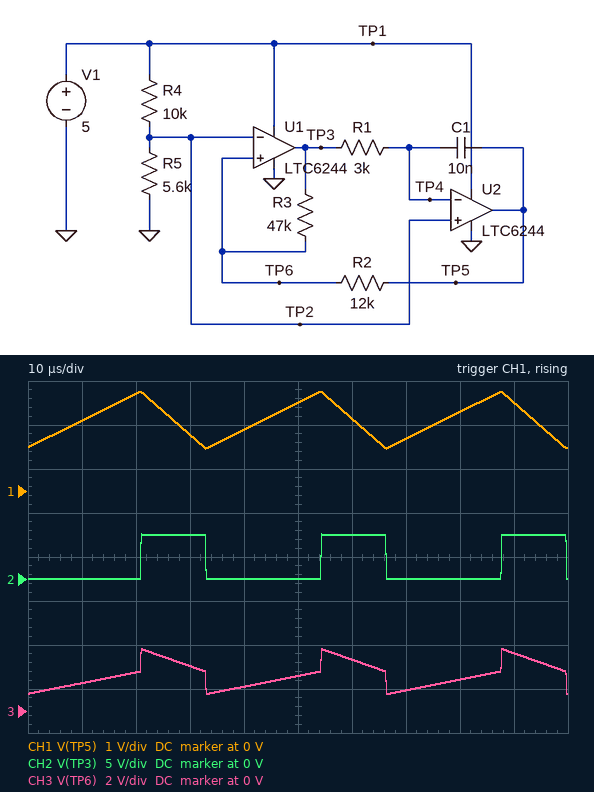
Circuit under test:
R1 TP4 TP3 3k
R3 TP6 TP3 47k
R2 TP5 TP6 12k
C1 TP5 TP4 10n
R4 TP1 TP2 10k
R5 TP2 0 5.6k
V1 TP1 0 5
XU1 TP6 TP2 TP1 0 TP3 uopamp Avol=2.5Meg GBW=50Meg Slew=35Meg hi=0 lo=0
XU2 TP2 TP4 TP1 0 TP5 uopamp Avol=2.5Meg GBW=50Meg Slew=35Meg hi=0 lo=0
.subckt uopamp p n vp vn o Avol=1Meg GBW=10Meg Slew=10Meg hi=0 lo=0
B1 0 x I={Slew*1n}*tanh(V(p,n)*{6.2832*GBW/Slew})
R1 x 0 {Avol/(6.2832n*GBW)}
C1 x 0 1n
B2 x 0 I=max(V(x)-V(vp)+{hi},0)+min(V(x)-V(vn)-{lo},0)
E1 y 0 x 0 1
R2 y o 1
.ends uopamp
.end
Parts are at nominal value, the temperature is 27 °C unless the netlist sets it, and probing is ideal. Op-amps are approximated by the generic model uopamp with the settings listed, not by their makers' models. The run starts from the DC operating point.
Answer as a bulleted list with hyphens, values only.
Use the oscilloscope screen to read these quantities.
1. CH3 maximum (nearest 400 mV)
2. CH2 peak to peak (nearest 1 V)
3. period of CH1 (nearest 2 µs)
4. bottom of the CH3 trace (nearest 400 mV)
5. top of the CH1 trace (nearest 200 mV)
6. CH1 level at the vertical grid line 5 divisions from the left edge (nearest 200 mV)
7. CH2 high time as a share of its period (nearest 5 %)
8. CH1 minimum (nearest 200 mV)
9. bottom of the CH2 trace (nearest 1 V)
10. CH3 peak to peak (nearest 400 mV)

- 2.8 V
- 5 V
- 34 µs
- 800 mV
- 2.2 V
- 2.0 V
- 35 %
- 1.0 V
- 0 V
- 2.0 V
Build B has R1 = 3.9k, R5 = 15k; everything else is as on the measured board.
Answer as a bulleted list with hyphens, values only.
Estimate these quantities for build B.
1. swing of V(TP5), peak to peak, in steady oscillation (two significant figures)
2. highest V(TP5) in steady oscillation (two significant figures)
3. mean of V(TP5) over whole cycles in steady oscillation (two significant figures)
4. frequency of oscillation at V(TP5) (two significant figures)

- 1.3 V
- 3.8 V
- 3.1 V
- 24 kHz
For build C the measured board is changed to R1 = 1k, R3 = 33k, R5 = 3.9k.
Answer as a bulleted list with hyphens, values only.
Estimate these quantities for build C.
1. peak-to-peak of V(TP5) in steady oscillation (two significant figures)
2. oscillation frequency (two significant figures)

- 1.9 V
- 55 kHz
